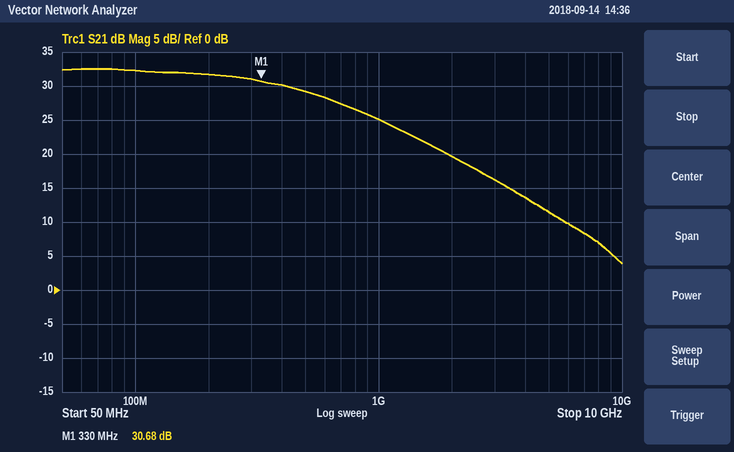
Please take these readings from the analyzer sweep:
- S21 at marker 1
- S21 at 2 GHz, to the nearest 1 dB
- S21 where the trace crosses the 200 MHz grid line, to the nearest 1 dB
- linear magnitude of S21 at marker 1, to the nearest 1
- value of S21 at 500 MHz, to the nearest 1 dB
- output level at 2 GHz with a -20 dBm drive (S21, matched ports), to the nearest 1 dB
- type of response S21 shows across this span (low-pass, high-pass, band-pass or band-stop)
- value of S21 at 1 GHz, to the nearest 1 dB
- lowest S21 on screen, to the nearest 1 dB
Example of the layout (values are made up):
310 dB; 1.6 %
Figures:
30.68 dB; 20 dB; 32 dB; 34; 29 dB; 0 dBm; low-pass; 25 dB; 4 dB
